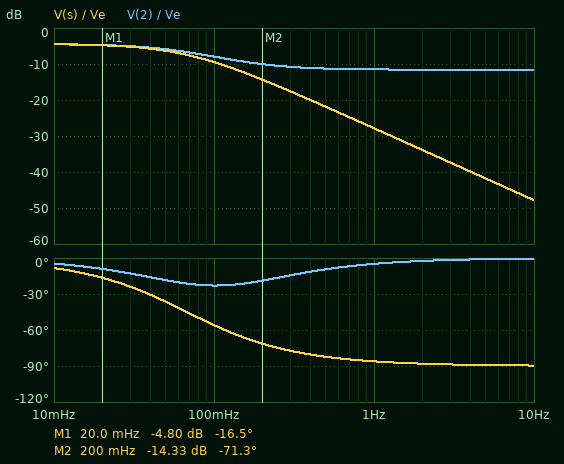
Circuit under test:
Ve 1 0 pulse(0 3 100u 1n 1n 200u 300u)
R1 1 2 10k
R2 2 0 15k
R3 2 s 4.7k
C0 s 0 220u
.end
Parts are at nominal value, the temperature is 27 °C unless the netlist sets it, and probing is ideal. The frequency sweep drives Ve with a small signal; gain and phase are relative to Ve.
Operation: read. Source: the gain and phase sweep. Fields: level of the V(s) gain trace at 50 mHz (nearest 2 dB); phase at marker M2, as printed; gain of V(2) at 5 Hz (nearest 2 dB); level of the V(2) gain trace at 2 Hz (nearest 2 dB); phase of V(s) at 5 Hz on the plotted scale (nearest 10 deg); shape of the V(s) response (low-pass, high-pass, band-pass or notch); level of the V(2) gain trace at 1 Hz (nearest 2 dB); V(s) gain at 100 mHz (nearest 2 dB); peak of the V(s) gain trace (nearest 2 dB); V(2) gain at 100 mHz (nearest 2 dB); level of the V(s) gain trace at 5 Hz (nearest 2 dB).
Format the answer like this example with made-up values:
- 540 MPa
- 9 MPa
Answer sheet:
- -6 dB
- -71.3 deg
- -12 dB
- -12 dB
- -90 deg
- low-pass
- -12 dB
- -10 dB
- -4 dB
- -8 dB
- -42 dB
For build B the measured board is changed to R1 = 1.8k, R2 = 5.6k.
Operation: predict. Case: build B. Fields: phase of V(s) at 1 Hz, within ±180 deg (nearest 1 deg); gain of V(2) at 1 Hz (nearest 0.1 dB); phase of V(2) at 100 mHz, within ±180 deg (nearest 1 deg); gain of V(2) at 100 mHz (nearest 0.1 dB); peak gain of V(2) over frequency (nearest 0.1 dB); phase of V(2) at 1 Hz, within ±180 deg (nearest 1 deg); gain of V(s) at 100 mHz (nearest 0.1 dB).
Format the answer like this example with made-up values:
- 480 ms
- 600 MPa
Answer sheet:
- -83 deg
- -4.6 dB
- -7 deg
- -3.2 dB
- -2.4 dB
- -2 deg
- -4.7 dB
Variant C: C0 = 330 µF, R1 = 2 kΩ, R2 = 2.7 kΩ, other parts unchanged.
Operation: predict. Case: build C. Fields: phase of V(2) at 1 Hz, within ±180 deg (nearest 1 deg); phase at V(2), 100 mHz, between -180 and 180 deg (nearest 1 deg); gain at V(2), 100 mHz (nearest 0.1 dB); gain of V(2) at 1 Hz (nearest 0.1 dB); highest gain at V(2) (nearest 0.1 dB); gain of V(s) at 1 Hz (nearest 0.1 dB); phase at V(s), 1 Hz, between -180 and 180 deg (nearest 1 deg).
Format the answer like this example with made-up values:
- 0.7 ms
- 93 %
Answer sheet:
- -1 deg
- -6 deg
- -5.8 dB
- -6.7 dB
- -4.8 dB
- -26.5 dB
- -85 deg
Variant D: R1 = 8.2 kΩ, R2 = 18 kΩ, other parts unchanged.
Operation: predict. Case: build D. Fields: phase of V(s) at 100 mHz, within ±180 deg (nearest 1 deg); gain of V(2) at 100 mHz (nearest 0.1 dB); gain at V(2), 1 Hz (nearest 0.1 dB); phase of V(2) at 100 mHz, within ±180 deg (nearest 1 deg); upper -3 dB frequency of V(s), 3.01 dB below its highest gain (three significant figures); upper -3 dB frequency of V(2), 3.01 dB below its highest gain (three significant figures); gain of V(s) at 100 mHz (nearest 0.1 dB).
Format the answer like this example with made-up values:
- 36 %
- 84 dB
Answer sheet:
- -55 deg
- -6.6 dB
- -10.0 dB
- -22 deg
- 70.0 mHz
- 91.4 mHz
- -8.1 dB
